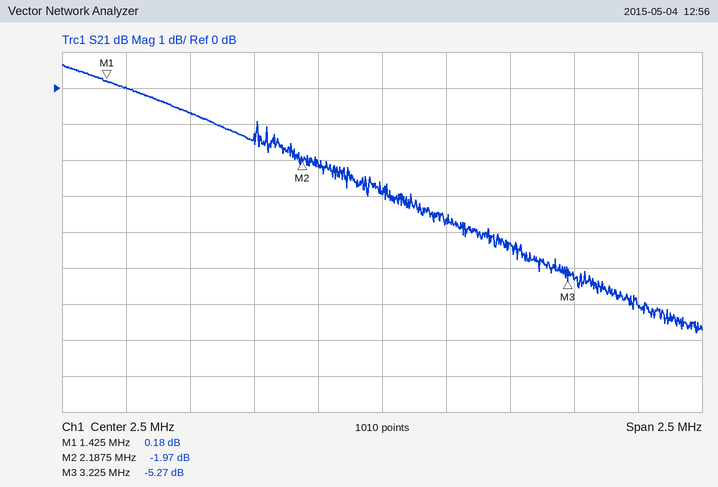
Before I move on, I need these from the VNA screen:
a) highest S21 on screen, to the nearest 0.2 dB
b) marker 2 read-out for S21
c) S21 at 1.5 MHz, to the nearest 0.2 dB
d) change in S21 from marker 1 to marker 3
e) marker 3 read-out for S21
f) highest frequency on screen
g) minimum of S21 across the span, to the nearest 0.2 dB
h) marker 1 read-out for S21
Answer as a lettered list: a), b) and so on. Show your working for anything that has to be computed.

a) 0.6 dB
b) -1.97 dB
c) 0.0 dB
d) -5.27 − (0.18) = -5.45 dB
e) -5.27 dB
f) 3.75 MHz
g) -6.8 dB
h) 0.18 dB
